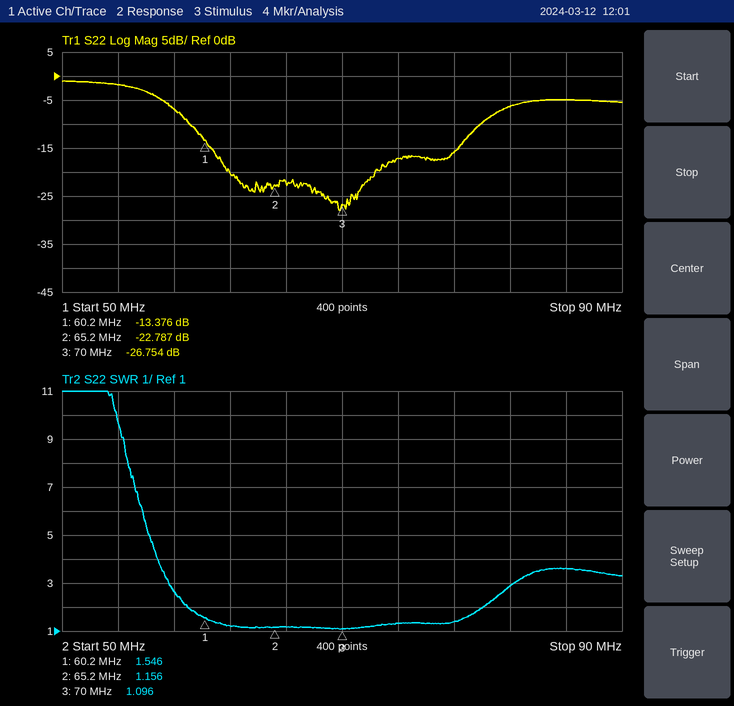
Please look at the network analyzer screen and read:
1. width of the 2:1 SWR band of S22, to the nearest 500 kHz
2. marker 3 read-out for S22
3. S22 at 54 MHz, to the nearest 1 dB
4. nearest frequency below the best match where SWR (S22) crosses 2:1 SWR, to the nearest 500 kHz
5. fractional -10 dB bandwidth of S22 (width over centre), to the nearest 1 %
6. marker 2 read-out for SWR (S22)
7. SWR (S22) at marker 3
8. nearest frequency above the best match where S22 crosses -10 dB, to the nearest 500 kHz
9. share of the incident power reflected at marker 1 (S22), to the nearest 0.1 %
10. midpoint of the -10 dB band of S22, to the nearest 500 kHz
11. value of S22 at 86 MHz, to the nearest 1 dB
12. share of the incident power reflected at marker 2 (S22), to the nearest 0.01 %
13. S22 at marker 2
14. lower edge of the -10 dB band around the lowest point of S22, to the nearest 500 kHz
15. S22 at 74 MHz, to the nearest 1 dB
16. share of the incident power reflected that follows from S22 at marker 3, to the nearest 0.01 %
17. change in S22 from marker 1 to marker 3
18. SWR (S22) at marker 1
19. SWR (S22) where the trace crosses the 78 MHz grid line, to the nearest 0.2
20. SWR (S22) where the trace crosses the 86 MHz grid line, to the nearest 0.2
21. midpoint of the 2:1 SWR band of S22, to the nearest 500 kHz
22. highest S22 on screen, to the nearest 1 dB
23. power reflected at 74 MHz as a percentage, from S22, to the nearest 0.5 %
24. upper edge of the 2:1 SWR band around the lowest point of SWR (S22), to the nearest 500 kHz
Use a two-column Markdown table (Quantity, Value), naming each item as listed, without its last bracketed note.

| Quantity | Value |
|---|---|
| width of the 2:1 SWR band of S22, to the nearest 500 kHz | 21.0 MHz |
| marker 3 read-out for S22 | -26.754 dB |
| S22 at 54 MHz, to the nearest 1 dB | -2 dB |
| nearest frequency below the best match where SWR (S22) crosses 2:1 SWR, to the nearest 500 kHz | 59.0 MHz |
| fractional -10 dB bandwidth of S22 (width over centre), to the nearest 1 % | 30 % |
| marker 2 read-out for SWR | 1.156 |
| SWR (S22) at marker 3 | 1.096 |
| nearest frequency above the best match where S22 crosses -10 dB, to the nearest 500 kHz | 80.0 MHz |
| share of the incident power reflected at marker 1 (S22), to the nearest 0.1 % | 4.6 % |
| midpoint of the -10 dB band of S22, to the nearest 500 kHz | 69.5 MHz |
| value of S22 at 86 MHz, to the nearest 1 dB | -5 dB |
| share of the incident power reflected at marker 2 (S22), to the nearest 0.01 % | 0.53 % |
| S22 at marker 2 | -22.787 dB |
| lower edge of the -10 dB band around the lowest point of S22, to the nearest 500 kHz | 59.0 MHz |
| S22 at 74 MHz, to the nearest 1 dB | -17 dB |
| share of the incident power reflected that follows from S22 at marker 3, to the nearest 0.01 % | 0.21 % |
| change in S22 from marker 1 to marker 3 | -13.378 dB |
| SWR (S22) at marker 1 | 1.546 |
| SWR (S22) where the trace crosses the 78 MHz grid line, to the nearest 0.2 | 1.4 |
| SWR (S22) where the trace crosses the 86 MHz grid line, to the nearest 0.2 | 3.6 |
| midpoint of the 2:1 SWR band of S22, to the nearest 500 kHz | 69.5 MHz |
| highest S22 on screen, to the nearest 1 dB | -1 dB |
| power reflected at 74 MHz as a percentage, from S22, to the nearest 0.5 % | 2.0 % |
| upper edge of the 2:1 SWR band around the lowest point of SWR (S22), to the nearest 500 kHz | 80.0 MHz |
